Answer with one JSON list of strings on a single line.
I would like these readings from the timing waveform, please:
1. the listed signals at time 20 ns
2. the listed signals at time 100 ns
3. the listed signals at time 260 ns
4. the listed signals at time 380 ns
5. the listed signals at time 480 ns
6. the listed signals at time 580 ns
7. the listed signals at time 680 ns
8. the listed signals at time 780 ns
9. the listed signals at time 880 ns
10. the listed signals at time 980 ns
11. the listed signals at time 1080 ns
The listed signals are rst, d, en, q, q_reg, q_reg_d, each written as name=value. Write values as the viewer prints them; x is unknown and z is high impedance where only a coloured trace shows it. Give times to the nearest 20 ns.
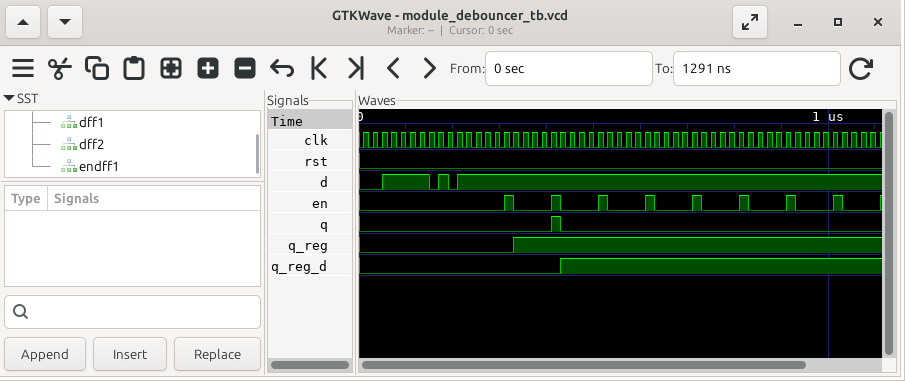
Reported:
["rst=0, d=0, en=0, q=0, q_reg=0, q_reg_d=0", "rst=0, d=1, en=0, q=0, q_reg=0, q_reg_d=0", "rst=0, d=1, en=0, q=0, q_reg=0, q_reg_d=0", "rst=0, d=1, en=0, q=0, q_reg=1, q_reg_d=0", "rst=0, d=1, en=0, q=0, q_reg=1, q_reg_d=1", "rst=0, d=1, en=0, q=0, q_reg=1, q_reg_d=1", "rst=0, d=1, en=0, q=0, q_reg=1, q_reg_d=1", "rst=0, d=1, en=0, q=0, q_reg=1, q_reg_d=1", "rst=0, d=1, en=0, q=0, q_reg=1, q_reg_d=1", "rst=0, d=1, en=0, q=0, q_reg=1, q_reg_d=1", "rst=0, d=1, en=0, q=0, q_reg=1, q_reg_d=1"]
